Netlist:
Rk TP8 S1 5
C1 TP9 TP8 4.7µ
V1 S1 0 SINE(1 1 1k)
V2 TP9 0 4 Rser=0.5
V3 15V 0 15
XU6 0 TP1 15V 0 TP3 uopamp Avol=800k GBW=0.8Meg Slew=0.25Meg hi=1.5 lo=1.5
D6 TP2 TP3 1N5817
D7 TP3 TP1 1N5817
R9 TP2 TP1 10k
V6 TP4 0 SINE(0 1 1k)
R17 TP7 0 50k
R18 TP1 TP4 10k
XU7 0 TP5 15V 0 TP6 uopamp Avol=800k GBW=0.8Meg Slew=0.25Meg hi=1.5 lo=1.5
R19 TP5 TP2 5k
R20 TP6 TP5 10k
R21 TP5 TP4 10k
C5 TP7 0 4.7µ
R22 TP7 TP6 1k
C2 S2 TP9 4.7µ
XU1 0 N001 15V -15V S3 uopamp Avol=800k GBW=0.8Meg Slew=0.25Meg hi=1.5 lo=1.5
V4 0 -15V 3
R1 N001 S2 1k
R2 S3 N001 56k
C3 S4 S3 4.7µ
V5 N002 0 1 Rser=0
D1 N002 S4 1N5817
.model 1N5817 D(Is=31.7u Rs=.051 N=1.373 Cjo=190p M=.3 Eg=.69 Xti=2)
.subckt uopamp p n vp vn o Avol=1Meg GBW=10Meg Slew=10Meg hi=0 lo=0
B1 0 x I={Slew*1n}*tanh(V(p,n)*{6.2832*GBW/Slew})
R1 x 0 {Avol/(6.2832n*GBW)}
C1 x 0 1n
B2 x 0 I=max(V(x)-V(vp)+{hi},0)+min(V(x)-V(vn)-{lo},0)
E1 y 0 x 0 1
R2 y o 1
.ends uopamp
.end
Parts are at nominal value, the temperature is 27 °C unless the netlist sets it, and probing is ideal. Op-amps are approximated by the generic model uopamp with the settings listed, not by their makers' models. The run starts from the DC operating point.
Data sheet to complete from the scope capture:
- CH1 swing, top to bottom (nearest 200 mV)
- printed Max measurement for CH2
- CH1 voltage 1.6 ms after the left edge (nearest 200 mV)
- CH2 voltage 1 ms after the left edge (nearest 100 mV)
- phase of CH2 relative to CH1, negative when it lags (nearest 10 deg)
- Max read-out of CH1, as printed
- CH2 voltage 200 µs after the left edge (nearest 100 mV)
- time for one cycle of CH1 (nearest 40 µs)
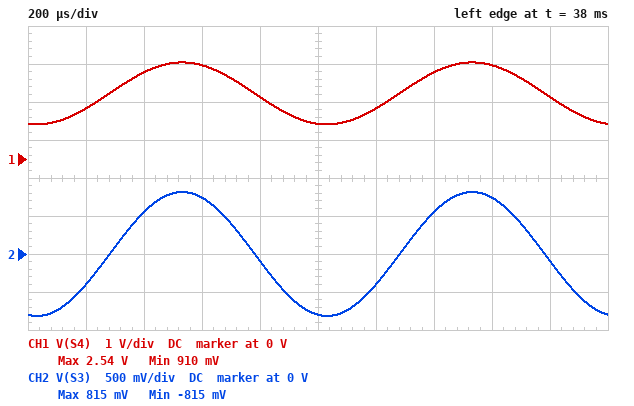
1.6 V
815 mV
2.4 V
-800 mV
0 deg
2.54 V
-400 mV
1.00 ms
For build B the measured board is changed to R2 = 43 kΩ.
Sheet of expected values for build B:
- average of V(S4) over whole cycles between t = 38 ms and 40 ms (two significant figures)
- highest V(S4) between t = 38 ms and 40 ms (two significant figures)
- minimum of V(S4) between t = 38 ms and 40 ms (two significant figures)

1.5 V
2.2 V
920 mV
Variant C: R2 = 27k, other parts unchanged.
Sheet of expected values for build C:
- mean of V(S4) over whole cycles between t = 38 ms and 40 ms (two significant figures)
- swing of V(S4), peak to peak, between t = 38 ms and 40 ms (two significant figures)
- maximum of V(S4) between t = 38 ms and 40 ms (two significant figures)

1.3 V
790 mV
1.7 V
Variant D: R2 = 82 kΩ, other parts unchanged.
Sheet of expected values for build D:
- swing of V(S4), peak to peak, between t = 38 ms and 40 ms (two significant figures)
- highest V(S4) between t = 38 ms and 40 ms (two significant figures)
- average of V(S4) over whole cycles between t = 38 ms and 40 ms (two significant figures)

2.4 V
3.3 V
2.1 V
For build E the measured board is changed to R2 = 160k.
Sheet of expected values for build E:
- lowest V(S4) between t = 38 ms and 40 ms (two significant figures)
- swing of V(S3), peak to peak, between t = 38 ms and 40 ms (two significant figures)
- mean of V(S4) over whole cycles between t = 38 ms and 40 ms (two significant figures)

950 mV
3.6 V
2.5 V
